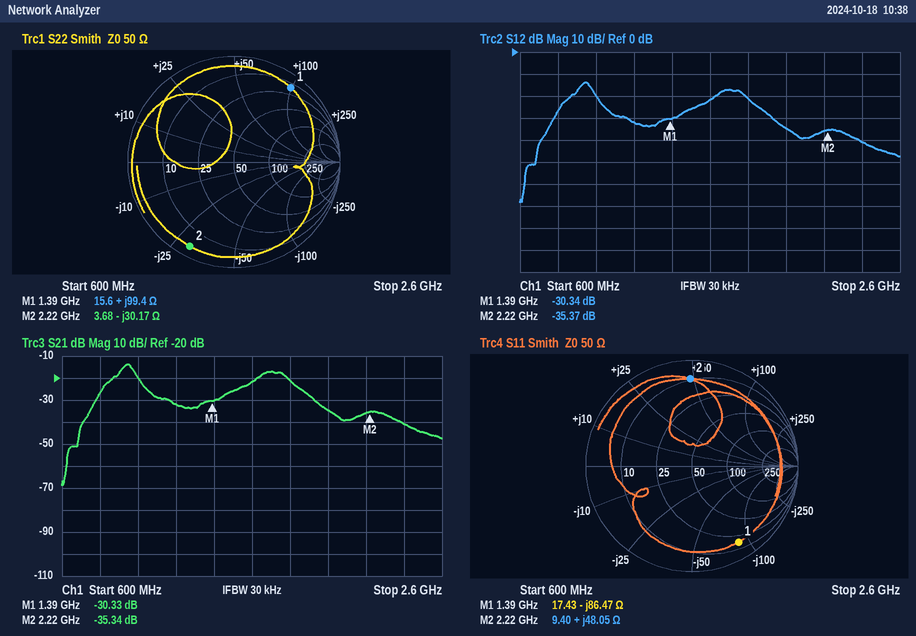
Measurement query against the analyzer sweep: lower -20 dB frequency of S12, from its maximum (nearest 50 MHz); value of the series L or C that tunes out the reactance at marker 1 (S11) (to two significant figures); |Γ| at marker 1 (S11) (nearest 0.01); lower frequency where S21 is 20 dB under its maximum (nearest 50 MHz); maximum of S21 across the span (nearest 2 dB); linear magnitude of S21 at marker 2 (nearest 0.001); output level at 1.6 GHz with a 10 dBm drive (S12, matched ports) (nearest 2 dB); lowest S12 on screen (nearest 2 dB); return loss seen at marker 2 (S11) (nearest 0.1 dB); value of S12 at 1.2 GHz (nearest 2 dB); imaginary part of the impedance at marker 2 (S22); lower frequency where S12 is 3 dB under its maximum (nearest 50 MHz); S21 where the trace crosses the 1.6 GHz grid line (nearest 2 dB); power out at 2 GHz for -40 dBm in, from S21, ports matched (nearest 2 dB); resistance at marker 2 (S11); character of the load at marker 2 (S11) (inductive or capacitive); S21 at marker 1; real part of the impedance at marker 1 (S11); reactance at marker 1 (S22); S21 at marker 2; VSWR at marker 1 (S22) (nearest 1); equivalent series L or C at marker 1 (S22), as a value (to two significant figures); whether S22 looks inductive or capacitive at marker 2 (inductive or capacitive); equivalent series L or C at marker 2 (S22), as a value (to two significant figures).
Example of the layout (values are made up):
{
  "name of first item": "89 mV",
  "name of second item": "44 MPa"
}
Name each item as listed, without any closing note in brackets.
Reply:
{
  "lower -20 dB frequency of S12, from its maximum": "750 MHz",
  "value of the series L or C that tunes out the reactance at marker 1 (S11)": "9.9 nH",
  "|Γ| at marker 1 (S11)": "0.84",
  "lower frequency where S21 is 20 dB under its maximum": "750 MHz",
  "maximum of S21 across the span": "-14 dB",
  "linear magnitude of S21 at marker 2": "0.017",
  "output level at 1.6 GHz with a 10 dBm drive (S12, matched ports)": "-12 dBm",
  "lowest S12 on screen": "-68 dB",
  "return loss seen at marker 2 (S11)": "1.7 dB",
  "value of S12 at 1.2 GHz": "-32 dB",
  "imaginary part of the impedance at marker 2": "-30.17 Ω",
  "lower frequency where S12 is 3 dB under its maximum": "900 MHz",
  "S21 where the trace crosses the 1.6 GHz grid line": "-22 dB",
  "power out at 2 GHz for -40 dBm in, from S21, ports matched": "-74 dBm",
  "resistance at marker 2": "9.40 Ω",
  "character of the load at marker 2 (S11)": "inductive",
  "S21 at marker 1": "-30.33 dB",
  "real part of the impedance at marker 1": "17.43 Ω",
  "reactance at marker 1": "+99.4 Ω",
  "S21 at marker 2": "-35.34 dB",
  "VSWR at marker 1 (S22)": "16",
  "equivalent series L or C at marker 1 (S22), as a value": "11 nH",
  "whether S22 looks inductive or capacitive at marker 2": "capacitive",
  "equivalent series L or C at marker 2 (S22), as a value": "2.4 pF"
}
